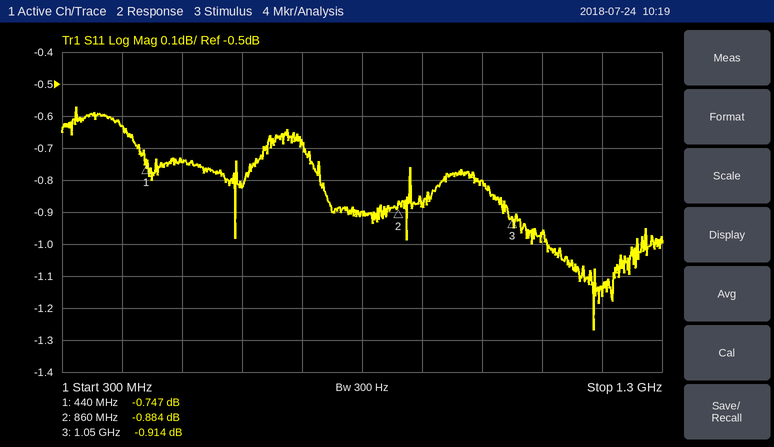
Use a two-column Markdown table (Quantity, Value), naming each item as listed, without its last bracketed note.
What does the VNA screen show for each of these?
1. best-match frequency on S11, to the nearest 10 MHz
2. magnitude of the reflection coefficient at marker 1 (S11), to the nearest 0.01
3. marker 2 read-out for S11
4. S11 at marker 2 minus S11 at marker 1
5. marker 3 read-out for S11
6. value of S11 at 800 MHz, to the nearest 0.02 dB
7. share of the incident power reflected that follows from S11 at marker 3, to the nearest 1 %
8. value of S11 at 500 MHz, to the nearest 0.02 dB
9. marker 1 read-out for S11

| Quantity | Value |
|---|---|
| best-match frequency on S11, to the nearest 10 MHz | 1.19 GHz |
| magnitude of the reflection coefficient at marker 1 (S11), to the nearest 0.01 | 0.92 |
| marker 2 read-out for S11 | -0.884 dB |
| S11 at marker 2 minus S11 at marker 1 | -0.137 dB |
| marker 3 read-out for S11 | -0.914 dB |
| value of S11 at 800 MHz, to the nearest 0.02 dB | -0.90 dB |
| share of the incident power reflected that follows from S11 at marker 3, to the nearest 1 % | 81 % |
| value of S11 at 500 MHz, to the nearest 0.02 dB | -0.74 dB |
| marker 1 read-out for S11 | -0.747 dB |
